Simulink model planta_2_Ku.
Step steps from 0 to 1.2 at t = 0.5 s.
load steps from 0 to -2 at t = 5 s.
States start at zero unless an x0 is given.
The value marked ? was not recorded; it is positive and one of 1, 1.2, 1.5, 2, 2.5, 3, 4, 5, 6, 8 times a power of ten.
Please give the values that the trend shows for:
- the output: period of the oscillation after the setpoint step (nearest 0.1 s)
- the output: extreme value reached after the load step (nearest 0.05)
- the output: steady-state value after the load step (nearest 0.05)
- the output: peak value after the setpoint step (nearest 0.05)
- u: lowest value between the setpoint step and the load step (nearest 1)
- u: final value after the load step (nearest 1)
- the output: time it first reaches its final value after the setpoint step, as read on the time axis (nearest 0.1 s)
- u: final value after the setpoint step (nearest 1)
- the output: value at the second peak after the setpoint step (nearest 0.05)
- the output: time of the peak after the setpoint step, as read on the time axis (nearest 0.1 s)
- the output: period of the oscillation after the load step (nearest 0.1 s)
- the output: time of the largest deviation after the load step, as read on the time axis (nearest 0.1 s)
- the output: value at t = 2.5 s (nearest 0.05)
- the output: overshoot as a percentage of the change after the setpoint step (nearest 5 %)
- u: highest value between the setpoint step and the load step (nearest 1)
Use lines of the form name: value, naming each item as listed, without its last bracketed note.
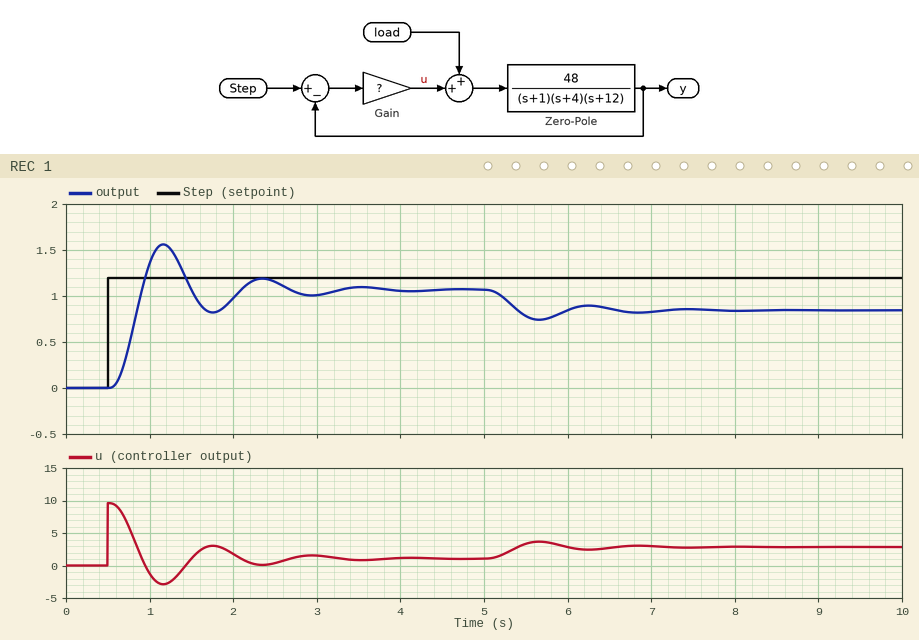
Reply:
the output: period of the oscillation after the setpoint step: 1.2 s
the output: extreme value reached after the load step: 0.75
the output: steady-state value after the load step: 0.85
the output: peak value after the setpoint step: 1.55
u: lowest value between the setpoint step and the load step: -3
u: final value after the load step: 3
the output: time it first reaches its final value after the setpoint step, as read on the time axis: 0.9 s
u: final value after the setpoint step: 1
the output: value at the second peak after the setpoint step: 1.20
the output: time of the peak after the setpoint step, as read on the time axis: 1.2 s
the output: period of the oscillation after the load step: 1.2 s
the output: time of the largest deviation after the load step, as read on the time axis: 5.7 s
the output: value at t = 2.5 s: 1.15
the output: overshoot as a percentage of the change after the setpoint step: 45 %
u: highest value between the setpoint step and the load step: 10
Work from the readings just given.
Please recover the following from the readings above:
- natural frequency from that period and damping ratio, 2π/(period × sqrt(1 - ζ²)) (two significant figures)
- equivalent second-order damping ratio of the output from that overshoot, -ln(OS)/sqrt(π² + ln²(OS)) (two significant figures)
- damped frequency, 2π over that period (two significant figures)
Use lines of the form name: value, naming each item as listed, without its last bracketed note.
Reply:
natural frequency from that period and damping ratio, 2π/(period × sqrt(1 - ζ²)): 5.4 rad/s
equivalent second-order damping ratio of the output from that overshoot, -ln(OS)/sqrt(π² + ln²(OS)): 0.25
damped frequency, 2π over that period: 5.2 rad/s
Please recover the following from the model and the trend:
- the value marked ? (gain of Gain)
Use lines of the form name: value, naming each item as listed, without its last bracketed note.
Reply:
the value marked ?: 8
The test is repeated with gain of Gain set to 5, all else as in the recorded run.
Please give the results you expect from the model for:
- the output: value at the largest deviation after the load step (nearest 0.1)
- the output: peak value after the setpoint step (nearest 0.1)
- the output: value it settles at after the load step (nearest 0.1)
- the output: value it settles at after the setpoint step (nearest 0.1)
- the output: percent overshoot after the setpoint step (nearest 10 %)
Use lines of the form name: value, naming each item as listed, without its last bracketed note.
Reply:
the output: value at the largest deviation after the load step: 0.6
the output: peak value after the setpoint step: 1.3
the output: value it settles at after the load step: 0.7
the output: value it settles at after the setpoint step: 1.0
the output: percent overshoot after the setpoint step: 30 %
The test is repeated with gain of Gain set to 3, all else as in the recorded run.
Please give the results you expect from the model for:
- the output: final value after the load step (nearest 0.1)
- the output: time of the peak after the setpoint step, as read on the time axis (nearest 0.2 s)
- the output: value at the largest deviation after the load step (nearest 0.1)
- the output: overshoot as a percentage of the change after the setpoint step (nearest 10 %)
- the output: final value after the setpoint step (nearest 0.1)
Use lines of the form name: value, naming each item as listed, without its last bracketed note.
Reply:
the output: final value after the load step: 0.4
the output: time of the peak after the setpoint step, as read on the time axis: 1.6 s
the output: value at the largest deviation after the load step: 0.3
the output: overshoot as a percentage of the change after the setpoint step: 20 %
the output: final value after the setpoint step: 0.9
